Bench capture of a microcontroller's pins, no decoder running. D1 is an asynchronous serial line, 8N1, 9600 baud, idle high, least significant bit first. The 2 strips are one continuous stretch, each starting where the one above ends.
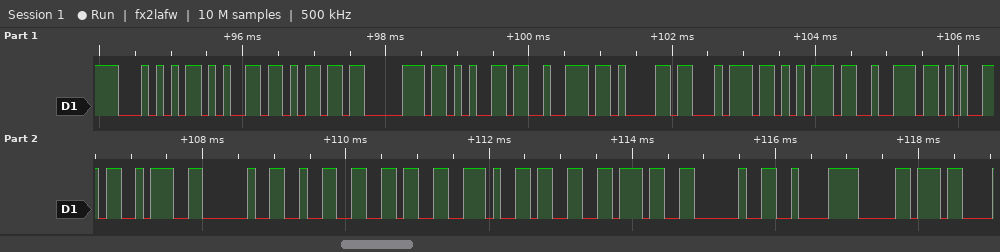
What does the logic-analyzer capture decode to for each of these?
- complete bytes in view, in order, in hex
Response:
0x54 0x65 0x6D 0x70 0x65 0x72 0x61 0x74 0x75 0x72 0x65 0x3A 0x20 0x32 0x36 0x2E 0x33 0x37 0x20 0xC2 0xB0
